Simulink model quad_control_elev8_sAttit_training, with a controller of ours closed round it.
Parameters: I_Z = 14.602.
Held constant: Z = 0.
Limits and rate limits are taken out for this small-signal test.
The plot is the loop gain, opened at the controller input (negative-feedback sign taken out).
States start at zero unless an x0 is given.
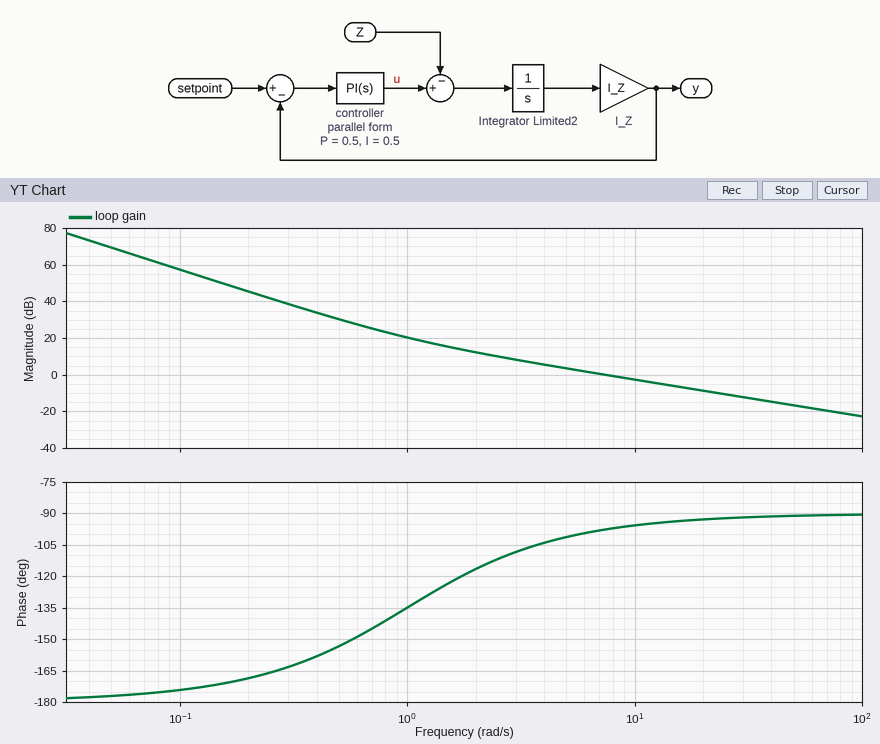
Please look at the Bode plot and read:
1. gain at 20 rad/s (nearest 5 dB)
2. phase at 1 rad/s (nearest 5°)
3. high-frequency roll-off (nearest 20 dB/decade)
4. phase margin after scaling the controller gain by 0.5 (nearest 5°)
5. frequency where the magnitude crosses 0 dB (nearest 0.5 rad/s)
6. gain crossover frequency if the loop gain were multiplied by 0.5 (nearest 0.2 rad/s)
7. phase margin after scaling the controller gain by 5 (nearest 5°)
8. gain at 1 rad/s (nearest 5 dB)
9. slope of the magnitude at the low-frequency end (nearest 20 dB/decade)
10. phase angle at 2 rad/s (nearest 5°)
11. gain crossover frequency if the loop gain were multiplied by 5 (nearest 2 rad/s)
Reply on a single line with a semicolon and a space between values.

-10 dB; -135°; -20 dB/decade; 75°; 7.5 rad/s; 3.8 rad/s; 90°; 20 dB; -40 dB/decade; -115°; 36 rad/s
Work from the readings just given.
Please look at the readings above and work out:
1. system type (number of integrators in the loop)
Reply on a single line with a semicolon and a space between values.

2
